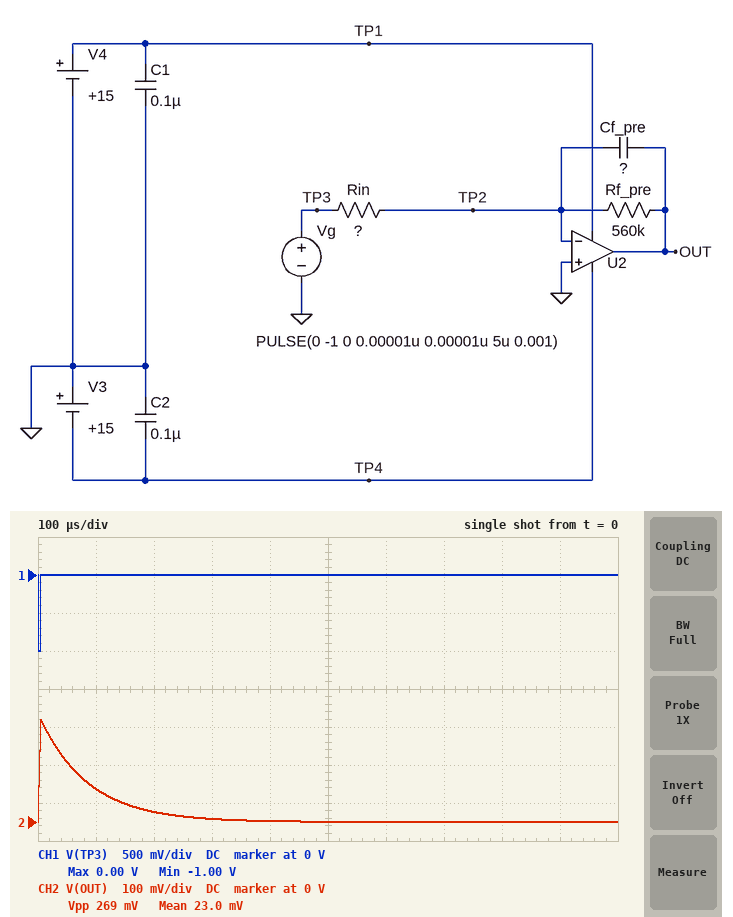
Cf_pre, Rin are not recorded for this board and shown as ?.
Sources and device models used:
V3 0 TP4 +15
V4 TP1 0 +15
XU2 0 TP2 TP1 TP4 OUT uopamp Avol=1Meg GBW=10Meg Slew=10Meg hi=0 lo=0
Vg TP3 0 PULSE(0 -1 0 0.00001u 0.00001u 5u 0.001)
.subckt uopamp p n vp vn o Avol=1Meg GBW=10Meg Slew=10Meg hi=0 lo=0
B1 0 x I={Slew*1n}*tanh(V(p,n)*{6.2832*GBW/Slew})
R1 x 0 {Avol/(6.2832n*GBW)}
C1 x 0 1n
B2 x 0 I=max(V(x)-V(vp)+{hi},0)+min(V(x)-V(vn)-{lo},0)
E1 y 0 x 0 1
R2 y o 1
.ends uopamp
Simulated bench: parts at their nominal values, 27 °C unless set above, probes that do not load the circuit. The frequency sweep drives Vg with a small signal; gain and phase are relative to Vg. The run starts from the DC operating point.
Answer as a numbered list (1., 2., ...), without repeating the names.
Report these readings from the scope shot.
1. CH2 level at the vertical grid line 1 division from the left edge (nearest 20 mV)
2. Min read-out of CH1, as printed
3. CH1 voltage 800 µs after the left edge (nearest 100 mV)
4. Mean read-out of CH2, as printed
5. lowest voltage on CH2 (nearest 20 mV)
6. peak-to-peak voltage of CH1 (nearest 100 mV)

1. 80 mV
2. -1.00 V
3. 0 V
4. 23.0 mV
5. 0 V
6. 1.0 V
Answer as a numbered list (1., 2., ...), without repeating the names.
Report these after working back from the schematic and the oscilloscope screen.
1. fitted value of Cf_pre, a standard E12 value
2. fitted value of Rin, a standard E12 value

1. 150 pF
2. 120 kΩ
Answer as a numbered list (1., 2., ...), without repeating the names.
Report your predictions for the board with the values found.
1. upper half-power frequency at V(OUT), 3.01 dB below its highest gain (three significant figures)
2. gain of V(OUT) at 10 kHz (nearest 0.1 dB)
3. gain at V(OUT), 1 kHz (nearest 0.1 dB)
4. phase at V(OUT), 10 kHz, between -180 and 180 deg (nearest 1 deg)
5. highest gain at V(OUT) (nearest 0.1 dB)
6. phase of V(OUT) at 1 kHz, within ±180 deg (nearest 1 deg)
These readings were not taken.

1. 1.89 kHz
2. -1.2 dB
3. 12.3 dB
4. 101 deg
5. 13.4 dB
6. 152 deg
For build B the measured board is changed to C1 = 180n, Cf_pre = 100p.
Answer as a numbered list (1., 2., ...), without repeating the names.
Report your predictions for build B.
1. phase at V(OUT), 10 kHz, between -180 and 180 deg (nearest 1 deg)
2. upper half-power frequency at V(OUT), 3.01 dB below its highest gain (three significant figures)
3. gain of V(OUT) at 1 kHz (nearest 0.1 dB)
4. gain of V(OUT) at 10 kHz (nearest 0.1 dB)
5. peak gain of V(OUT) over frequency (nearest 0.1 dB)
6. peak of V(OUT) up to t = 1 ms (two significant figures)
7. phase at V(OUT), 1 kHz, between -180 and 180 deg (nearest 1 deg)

1. 106 deg
2. 2.84 kHz
3. 12.9 dB
4. 2.1 dB
5. 13.4 dB
6. 400 mV
7. 161 deg
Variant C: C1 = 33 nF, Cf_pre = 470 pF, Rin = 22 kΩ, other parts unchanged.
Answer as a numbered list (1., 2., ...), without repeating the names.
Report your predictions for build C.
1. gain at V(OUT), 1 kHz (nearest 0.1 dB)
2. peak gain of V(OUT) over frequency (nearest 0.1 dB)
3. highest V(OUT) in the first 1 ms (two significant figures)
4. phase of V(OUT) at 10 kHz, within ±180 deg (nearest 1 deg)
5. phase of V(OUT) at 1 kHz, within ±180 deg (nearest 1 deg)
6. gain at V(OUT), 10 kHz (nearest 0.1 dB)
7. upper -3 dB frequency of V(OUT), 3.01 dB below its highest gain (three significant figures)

1. 22.4 dB
2. 28.1 dB
3. 480 mV
4. 93 deg
5. 121 deg
6. 3.7 dB
7. 604 Hz
